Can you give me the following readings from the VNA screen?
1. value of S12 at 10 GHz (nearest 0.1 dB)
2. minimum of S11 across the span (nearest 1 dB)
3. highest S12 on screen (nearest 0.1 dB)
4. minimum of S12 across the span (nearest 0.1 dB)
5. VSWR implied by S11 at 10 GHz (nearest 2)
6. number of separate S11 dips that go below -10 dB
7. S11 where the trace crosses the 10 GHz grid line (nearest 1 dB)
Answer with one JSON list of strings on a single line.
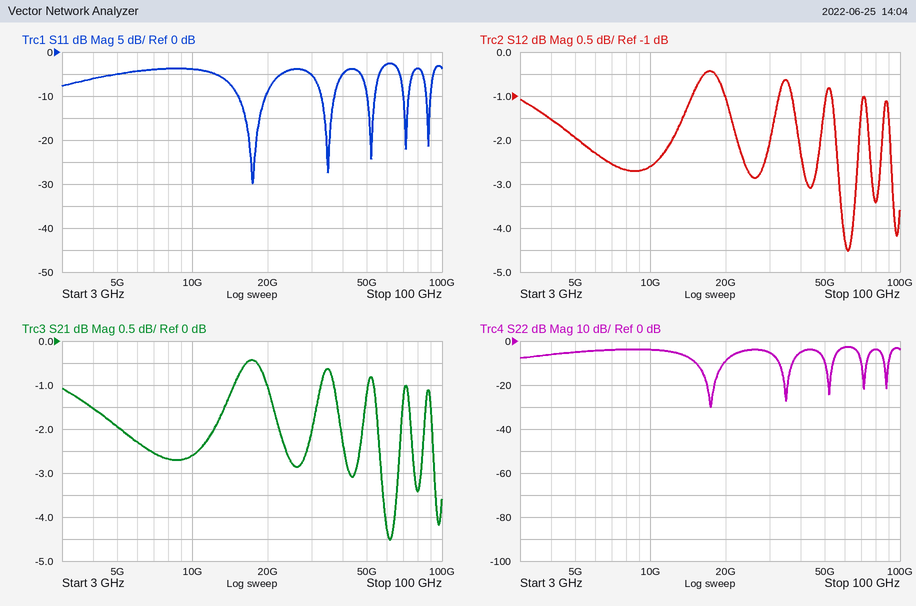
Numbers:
["-2.6 dB", "-30 dB", "-0.4 dB", "-4.5 dB", "4", "5", "-4 dB"]
